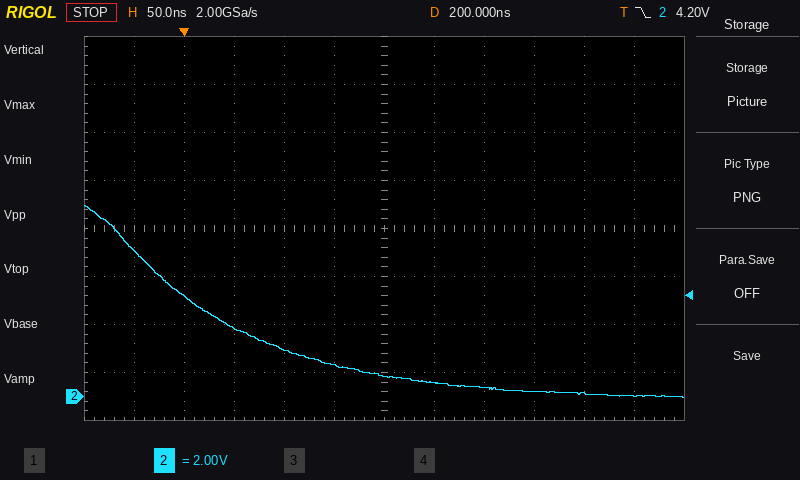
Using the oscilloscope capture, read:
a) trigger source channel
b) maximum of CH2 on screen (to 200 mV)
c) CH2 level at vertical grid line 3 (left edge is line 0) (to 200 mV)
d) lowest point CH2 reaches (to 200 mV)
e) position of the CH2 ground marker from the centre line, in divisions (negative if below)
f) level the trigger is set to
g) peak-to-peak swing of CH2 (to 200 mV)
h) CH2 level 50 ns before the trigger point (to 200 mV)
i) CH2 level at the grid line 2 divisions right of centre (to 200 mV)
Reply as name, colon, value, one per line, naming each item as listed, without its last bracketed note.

trigger source channel: CH2
maximum of CH2 on screen: 8.0 V
CH2 level at vertical grid line 3 (left edge is line 0): 2.8 V
lowest point CH2 reaches: 0.0 V
position of the CH2 ground marker from the centre line, in divisions: -3.5 div
level the trigger is set to: 4.20 V
peak-to-peak swing of CH2: 8.0 V
CH2 level 50 ns before the trigger point: 6.0 V
CH2 level at the grid line 2 divisions right of centre: 400 mV
